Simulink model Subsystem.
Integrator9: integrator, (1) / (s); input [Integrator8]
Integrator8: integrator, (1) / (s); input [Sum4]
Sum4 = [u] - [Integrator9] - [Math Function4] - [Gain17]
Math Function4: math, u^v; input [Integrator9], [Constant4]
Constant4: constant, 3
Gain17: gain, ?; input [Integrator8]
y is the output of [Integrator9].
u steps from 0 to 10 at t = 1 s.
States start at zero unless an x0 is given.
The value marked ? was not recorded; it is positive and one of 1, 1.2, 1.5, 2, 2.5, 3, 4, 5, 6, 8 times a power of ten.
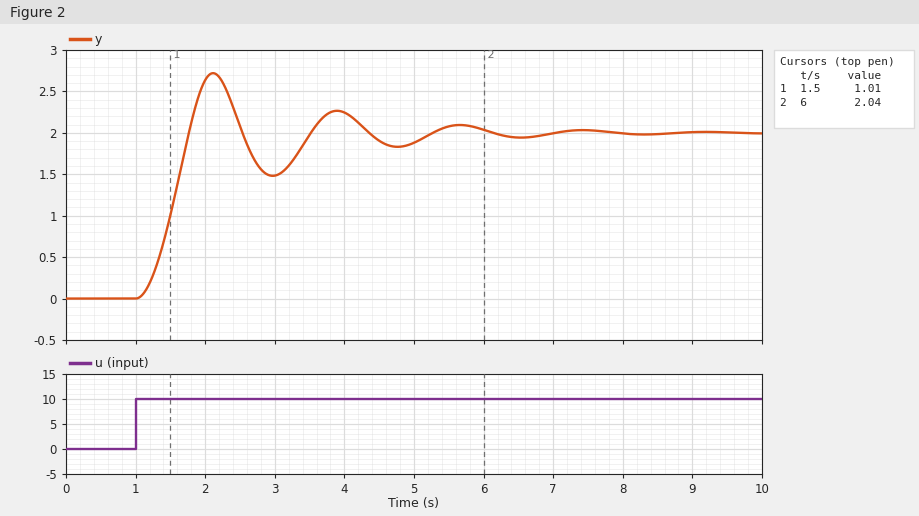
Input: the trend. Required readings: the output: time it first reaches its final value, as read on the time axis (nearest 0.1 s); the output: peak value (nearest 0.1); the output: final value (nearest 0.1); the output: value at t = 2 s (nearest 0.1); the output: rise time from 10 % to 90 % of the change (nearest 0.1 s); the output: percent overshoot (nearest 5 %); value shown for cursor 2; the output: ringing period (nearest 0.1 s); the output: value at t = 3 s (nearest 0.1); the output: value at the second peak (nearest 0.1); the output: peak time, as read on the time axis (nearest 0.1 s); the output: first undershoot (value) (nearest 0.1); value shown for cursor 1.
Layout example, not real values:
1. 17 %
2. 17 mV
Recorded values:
1. 1.8 s
2. 2.7
3. 2.0
4. 2.6
5. 0.5 s
6. 35 %
7. 2.04
8. 1.8 s
9. 1.5
10. 2.3
11. 2.1 s
12. 1.5
13. 1.01
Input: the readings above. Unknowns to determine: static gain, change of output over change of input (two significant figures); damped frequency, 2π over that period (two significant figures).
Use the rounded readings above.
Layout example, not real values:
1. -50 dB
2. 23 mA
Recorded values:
1. 0.20
2. 3.5 rad/s
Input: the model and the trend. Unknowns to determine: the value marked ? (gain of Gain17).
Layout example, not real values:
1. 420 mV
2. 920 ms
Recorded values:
1. 1.2
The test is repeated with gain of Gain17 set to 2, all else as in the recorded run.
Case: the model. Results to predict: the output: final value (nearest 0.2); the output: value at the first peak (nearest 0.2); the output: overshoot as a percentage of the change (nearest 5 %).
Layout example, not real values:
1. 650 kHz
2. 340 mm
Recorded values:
1. 2.0
2. 2.4
3. 25 %
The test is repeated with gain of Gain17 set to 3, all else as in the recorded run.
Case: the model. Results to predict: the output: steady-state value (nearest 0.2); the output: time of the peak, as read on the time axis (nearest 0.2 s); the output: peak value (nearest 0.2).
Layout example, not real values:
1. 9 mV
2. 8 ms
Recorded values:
1. 2.0
2. 2.4 s
3. 2.2
